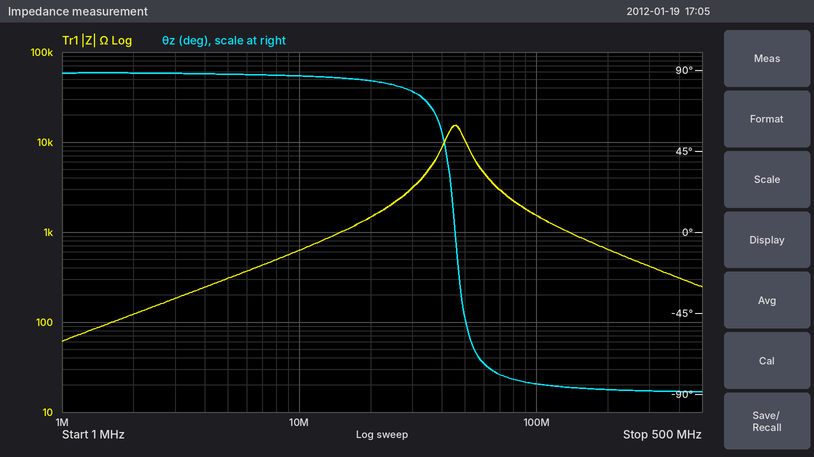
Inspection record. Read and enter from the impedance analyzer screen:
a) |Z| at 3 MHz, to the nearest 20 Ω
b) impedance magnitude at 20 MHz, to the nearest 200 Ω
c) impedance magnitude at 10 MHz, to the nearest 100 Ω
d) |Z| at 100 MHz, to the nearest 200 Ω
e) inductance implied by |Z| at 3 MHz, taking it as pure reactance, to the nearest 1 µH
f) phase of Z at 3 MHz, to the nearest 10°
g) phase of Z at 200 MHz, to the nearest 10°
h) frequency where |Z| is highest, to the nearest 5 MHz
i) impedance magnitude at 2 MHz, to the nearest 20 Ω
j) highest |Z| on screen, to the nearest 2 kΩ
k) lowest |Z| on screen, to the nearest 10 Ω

180 Ω
1.4 kΩ
600 Ω
1.6 kΩ
10 µH
90°
-90°
45 MHz
120 Ω
16 kΩ
60 Ω
